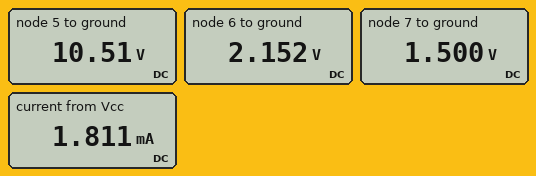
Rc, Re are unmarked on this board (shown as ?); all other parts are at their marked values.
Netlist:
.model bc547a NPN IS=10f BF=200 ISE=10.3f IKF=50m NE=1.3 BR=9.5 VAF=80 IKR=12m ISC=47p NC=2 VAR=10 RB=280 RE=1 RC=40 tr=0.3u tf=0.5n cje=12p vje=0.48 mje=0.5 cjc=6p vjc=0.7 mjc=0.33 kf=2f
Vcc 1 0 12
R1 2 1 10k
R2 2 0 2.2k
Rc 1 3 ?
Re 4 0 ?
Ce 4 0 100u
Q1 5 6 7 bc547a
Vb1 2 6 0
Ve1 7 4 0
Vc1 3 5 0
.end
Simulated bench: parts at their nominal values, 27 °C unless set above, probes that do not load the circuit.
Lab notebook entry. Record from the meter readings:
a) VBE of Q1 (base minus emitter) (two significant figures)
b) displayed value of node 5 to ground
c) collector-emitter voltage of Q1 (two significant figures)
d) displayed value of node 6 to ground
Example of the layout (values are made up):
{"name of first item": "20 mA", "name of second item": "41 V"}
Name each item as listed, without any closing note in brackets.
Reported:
{"VBE of Q1 (base minus emitter)": "650 mV", "displayed value of node 5 to ground": "10.51 V", "collector-emitter voltage of Q1": "9.0 V", "displayed value of node 6 to ground": "2.152 V"}
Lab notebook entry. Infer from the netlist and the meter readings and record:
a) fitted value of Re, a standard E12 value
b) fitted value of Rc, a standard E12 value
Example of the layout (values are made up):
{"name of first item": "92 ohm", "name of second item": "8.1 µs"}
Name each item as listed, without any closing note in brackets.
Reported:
{"fitted value of Re, a standard E12 value": "1.8 kΩ", "fitted value of Rc, a standard E12 value": "1.8 kΩ"}
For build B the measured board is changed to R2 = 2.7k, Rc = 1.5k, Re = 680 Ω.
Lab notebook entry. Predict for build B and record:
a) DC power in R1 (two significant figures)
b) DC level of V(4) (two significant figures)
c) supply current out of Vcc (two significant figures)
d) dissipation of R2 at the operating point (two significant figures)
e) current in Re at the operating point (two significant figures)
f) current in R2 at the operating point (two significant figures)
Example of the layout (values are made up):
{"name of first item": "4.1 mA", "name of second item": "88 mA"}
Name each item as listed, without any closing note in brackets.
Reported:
{"DC power in R1": "9.0 mW", "DC level of V(4)": "1.8 V", "supply current out of Vcc": "3.6 mA", "dissipation of R2 at the operating point": "2.3 mW", "current in Re at the operating point": "2.7 mA", "current in R2 at the operating point": "930 µA"}
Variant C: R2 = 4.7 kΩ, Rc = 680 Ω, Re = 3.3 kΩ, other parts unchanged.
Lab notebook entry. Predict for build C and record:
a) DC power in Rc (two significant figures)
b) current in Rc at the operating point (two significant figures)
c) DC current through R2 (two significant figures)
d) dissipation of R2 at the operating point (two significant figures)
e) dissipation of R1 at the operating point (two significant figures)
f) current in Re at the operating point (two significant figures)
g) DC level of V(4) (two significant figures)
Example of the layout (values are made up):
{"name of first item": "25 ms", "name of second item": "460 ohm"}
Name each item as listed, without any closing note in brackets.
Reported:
{"DC power in Rc": "610 µW", "current in Rc at the operating point": "950 µA", "DC current through R2": "810 µA", "dissipation of R2 at the operating point": "3.1 mW", "dissipation of R1 at the operating point": "6.7 mW", "current in Re at the operating point": "960 µA", "DC level of V(4)": "3.2 V"}
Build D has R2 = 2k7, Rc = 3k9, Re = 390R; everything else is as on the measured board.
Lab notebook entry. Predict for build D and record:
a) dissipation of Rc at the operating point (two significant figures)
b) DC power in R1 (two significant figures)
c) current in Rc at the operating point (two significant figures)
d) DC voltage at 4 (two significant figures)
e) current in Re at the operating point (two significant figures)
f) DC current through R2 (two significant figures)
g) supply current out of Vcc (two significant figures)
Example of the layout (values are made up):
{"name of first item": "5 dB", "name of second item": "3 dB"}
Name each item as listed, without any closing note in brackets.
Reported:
{"dissipation of Rc at the operating point": "29 mW", "DC power in R1": "10 mW", "current in Rc at the operating point": "2.7 mA", "DC voltage at 4": "1.2 V", "current in Re at the operating point": "3.0 mA", "DC current through R2": "730 µA", "supply current out of Vcc": "3.7 mA"}
